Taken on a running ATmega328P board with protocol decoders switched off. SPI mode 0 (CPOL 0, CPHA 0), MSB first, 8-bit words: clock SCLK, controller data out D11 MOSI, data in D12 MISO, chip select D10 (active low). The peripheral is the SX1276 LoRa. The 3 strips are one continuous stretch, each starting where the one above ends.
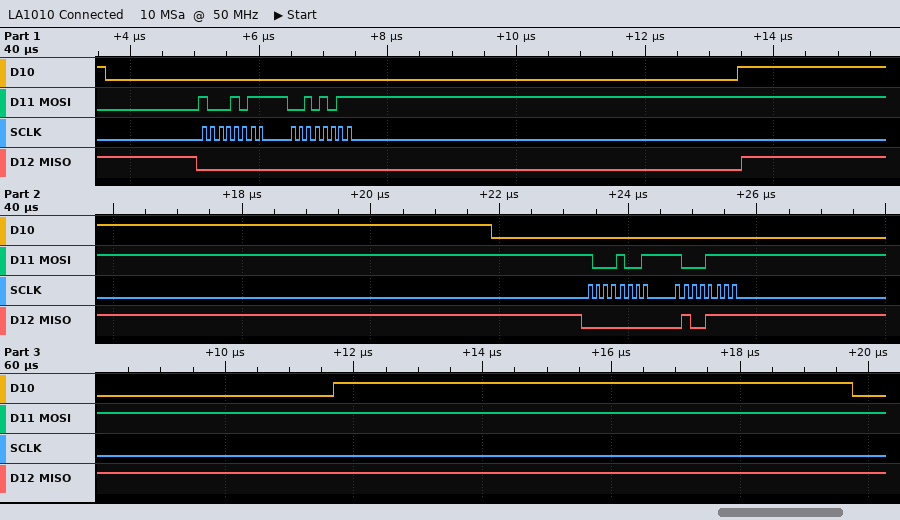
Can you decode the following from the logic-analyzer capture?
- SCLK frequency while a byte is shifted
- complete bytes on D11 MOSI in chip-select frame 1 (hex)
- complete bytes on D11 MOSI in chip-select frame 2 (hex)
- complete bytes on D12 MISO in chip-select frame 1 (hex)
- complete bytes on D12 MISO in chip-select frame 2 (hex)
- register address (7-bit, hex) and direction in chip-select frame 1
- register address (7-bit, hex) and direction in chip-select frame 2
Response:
8 MHz
8B 2B
89 8F
00 00
00 4F
0x0B write
0x09 write
